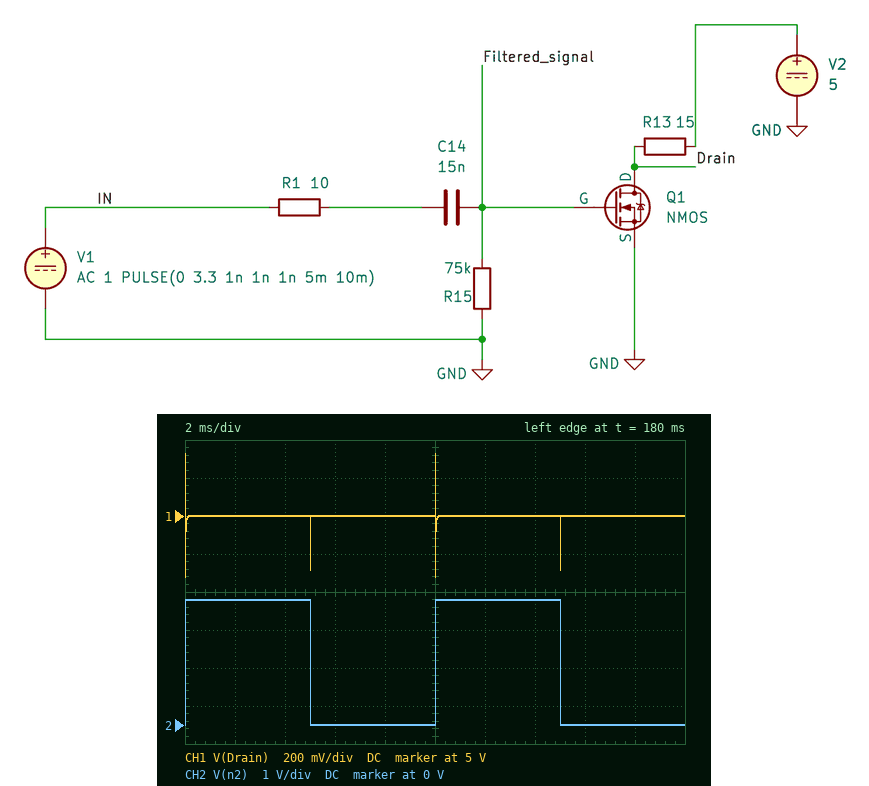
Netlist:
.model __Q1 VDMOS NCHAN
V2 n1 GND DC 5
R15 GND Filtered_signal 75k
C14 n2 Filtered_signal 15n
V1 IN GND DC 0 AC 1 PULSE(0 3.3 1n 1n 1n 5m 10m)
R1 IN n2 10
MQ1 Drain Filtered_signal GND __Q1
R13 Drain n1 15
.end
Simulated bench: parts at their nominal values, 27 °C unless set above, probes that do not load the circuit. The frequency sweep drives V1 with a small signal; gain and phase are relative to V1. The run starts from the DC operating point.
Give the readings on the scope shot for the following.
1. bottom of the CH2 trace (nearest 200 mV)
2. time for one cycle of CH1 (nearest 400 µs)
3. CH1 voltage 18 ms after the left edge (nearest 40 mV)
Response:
0 V
10.0 ms
5.00 V
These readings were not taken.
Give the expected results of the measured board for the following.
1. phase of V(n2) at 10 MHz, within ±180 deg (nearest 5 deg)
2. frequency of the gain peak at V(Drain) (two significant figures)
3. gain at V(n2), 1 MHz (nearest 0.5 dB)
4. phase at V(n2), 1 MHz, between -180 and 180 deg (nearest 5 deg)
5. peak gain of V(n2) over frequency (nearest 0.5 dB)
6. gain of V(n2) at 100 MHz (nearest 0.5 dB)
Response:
-40 deg
19 MHz
0 dB
-5 deg
0 dB
-18.5 dB
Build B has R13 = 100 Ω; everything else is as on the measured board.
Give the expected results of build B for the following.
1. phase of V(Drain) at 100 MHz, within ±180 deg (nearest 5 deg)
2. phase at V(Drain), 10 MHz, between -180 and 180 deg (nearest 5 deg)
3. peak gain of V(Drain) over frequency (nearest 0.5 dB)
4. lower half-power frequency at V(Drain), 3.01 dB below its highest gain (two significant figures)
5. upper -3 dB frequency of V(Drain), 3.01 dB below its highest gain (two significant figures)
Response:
-80 deg
-15 deg
-10.0 dB
2.7 MHz
19 MHz
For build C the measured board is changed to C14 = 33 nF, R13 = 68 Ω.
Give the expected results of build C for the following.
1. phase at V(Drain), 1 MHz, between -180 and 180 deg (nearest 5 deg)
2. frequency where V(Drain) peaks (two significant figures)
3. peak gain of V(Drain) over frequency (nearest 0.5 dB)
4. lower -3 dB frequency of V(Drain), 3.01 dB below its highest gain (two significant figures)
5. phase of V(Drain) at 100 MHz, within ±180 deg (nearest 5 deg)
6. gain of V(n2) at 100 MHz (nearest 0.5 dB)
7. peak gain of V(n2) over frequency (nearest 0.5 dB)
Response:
75 deg
8.6 MHz
-11.0 dB
3.4 MHz
-80 deg
-19.0 dB
0 dB
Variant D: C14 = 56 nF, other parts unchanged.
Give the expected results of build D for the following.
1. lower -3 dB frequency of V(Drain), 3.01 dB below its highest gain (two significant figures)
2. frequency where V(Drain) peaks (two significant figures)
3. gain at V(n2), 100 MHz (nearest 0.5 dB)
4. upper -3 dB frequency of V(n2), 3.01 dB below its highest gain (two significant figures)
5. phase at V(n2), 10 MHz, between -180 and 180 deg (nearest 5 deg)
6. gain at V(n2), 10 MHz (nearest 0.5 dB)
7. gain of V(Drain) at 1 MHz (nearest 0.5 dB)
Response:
6.7 MHz
18 MHz
-19.5 dB
10 MHz
-45 deg
-3.0 dB
-36.0 dB
